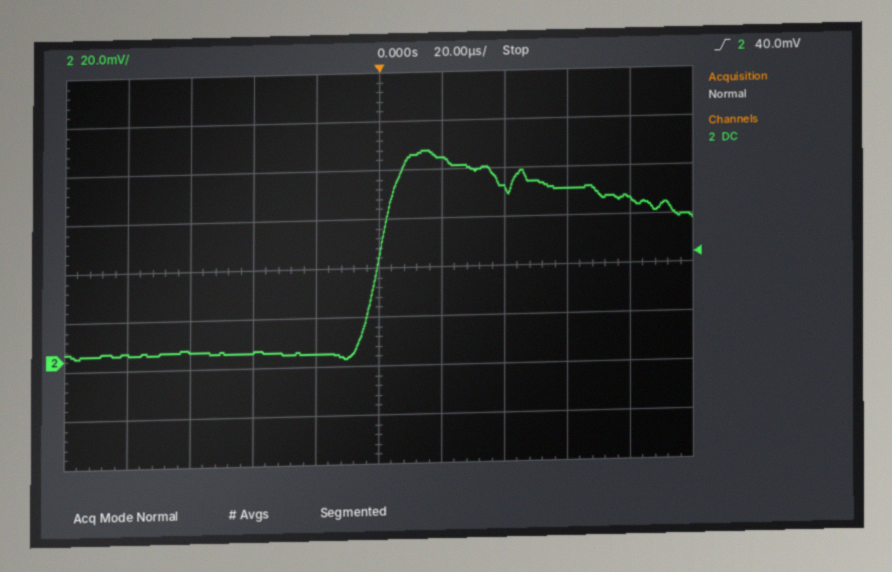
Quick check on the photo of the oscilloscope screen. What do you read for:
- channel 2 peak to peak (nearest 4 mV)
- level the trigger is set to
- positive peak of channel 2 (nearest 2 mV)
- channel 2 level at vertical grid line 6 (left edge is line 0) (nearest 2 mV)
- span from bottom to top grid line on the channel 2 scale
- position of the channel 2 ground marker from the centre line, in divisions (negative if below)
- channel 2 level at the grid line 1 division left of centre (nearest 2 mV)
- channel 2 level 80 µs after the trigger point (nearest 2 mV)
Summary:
84 mV
40.0 mV
84 mV
80 mV
160 mV
-1.8 div
2 mV
62 mV
